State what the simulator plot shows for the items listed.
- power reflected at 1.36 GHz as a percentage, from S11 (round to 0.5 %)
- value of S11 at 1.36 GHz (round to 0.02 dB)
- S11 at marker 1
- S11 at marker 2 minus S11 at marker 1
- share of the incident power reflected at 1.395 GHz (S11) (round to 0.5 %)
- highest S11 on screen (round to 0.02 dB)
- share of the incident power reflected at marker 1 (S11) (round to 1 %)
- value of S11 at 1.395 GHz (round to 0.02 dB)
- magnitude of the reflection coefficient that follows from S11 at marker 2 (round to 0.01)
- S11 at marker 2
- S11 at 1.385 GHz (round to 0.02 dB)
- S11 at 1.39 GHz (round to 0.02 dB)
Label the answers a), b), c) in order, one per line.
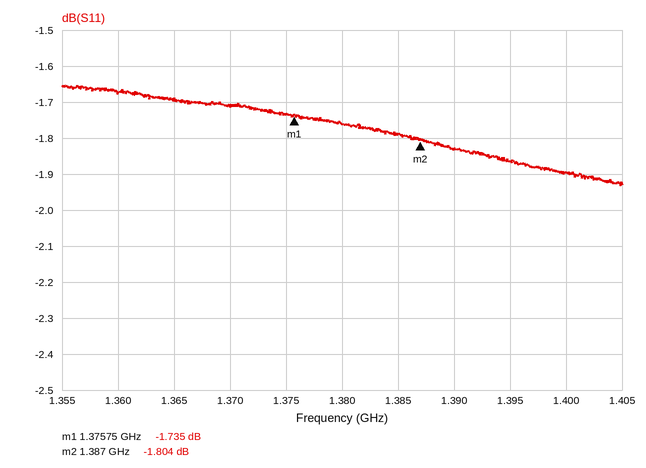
a) 68.0 %
b) -1.68 dB
c) -1.735 dB
d) -0.069 dB
e) 65.0 %
f) -1.66 dB
g) 67 %
h) -1.86 dB
i) 0.81
j) -1.804 dB
k) -1.78 dB
l) -1.82 dB
